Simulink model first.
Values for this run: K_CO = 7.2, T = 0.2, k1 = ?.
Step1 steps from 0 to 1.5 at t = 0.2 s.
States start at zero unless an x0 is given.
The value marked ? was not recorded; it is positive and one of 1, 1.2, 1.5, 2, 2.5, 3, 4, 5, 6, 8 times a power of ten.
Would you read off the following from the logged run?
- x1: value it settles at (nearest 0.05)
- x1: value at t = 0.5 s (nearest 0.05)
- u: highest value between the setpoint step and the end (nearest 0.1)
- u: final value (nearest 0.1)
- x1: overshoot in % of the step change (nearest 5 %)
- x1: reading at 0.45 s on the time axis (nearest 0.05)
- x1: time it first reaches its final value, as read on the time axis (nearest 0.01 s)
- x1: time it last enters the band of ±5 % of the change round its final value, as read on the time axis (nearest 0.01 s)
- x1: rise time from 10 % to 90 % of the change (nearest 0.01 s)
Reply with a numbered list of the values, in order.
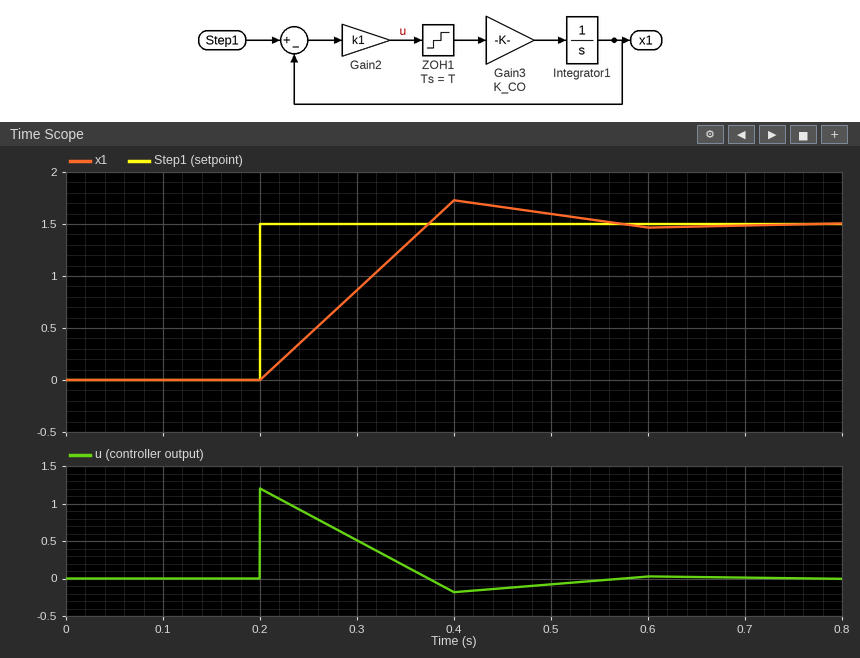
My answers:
1. 1.50
2. 1.60
3. 1.2
4. 0.0
5. 15 %
6. 1.65
7. 0.37 s
8. 0.52 s
9. 0.14 s
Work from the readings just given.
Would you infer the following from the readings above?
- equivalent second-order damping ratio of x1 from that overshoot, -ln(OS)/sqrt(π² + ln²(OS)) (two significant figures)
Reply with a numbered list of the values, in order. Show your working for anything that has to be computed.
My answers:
1. ln(0.15) = -1.897; 1.897 / sqrt(9.870 + 3.599) = 0.52
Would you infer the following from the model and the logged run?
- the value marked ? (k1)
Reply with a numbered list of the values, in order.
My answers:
1. 0.8
